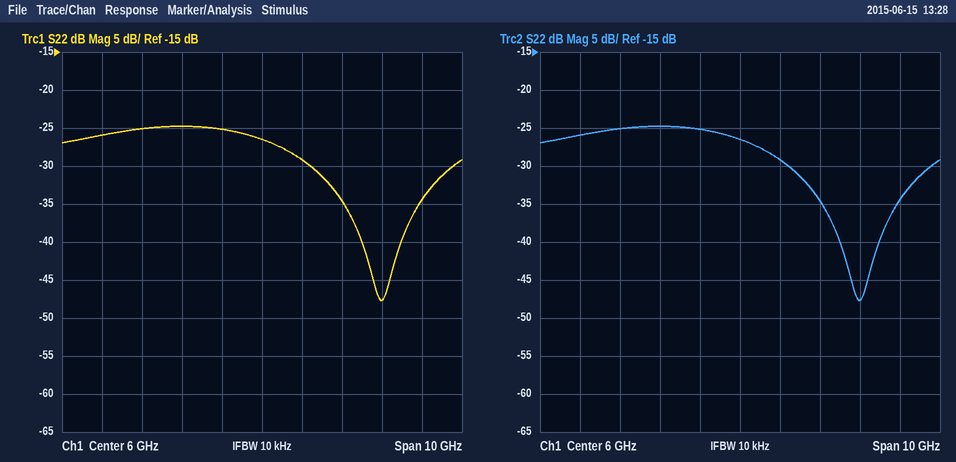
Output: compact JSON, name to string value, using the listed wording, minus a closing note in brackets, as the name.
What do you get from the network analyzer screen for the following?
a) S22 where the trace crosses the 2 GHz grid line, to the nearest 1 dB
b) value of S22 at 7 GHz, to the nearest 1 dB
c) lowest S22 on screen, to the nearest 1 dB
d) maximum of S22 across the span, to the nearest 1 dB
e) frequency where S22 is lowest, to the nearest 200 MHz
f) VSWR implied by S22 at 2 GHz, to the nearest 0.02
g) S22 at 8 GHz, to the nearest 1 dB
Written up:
{"S22 where the trace crosses the 2 GHz grid line, to the nearest 1 dB": "-26 dB", "value of S22 at 7 GHz, to the nearest 1 dB": "-29 dB", "lowest S22 on screen, to the nearest 1 dB": "-48 dB", "maximum of S22 across the span, to the nearest 1 dB": "-25 dB", "frequency where S22 is lowest, to the nearest 200 MHz": "9.0 GHz", "VSWR implied by S22 at 2 GHz, to the nearest 0.02": "1.10", "S22 at 8 GHz, to the nearest 1 dB": "-35 dB"}
